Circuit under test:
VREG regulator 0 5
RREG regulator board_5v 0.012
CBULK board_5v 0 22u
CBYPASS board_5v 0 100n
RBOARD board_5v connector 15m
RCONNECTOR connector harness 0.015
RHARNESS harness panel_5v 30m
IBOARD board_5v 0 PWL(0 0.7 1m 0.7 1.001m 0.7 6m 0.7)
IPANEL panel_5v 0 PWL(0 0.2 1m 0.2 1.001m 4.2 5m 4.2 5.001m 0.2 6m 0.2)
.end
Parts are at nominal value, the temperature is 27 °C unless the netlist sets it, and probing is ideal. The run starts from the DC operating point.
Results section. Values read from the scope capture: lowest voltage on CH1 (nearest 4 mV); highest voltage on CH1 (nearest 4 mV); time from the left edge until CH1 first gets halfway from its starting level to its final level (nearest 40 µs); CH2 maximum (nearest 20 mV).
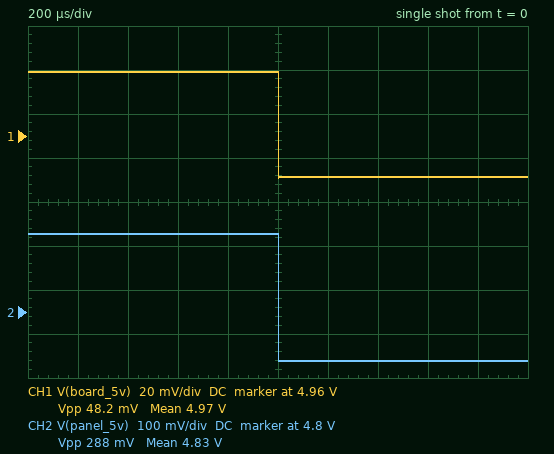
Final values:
4.940 V
4.988 V
1.00 ms
4.98 V
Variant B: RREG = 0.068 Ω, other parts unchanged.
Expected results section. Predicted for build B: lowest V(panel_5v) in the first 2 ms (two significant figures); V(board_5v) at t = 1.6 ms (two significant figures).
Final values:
4.4 V
4.7 V
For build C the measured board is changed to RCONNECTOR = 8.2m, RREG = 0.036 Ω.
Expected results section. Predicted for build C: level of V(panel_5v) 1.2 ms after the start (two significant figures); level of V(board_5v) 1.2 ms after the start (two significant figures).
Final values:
4.6 V
4.8 V
